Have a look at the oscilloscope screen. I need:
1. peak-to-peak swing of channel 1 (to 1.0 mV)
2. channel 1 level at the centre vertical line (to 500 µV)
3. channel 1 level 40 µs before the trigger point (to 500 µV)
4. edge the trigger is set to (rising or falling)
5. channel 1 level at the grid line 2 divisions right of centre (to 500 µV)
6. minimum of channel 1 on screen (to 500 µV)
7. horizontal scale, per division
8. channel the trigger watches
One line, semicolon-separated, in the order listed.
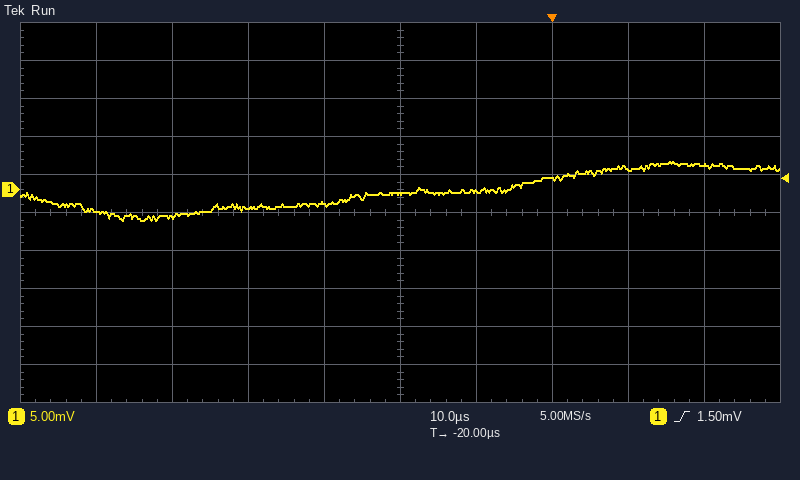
8.0 mV; -500 µV; -2.5 mV; rising; 1.5 mV; -4.0 mV; 10 µs; channel 1
